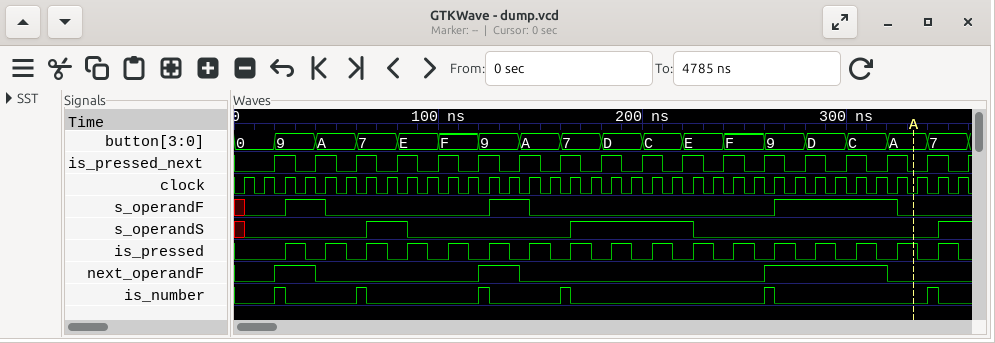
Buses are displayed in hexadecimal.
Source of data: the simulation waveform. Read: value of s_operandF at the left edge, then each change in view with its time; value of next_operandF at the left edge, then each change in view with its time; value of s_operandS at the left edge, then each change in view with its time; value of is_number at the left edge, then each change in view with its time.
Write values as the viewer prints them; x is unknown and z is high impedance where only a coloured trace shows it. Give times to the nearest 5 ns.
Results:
x, 0 at 5 ns, 1 at 25 ns, 0 at 45 ns, 1 at 125 ns, 0 at 145 ns, 1 at 265 ns, 0 at 325 ns
0, 1 at 20 ns, 0 at 40 ns, 1 at 120 ns, 0 at 140 ns, 1 at 260 ns, 0 at 320 ns
x, 0 at 5 ns, 1 at 65 ns, 0 at 85 ns, 1 at 165 ns, 0 at 225 ns, 1 at 345 ns
0, 1 at 20 ns, 0 at 25 ns, 1 at 60 ns, 0 at 65 ns, 1 at 120 ns, 0 at 125 ns, 1 at 160 ns, 0 at 165 ns, 1 at 260 ns, 0 at 265 ns, 1 at 340 ns, 0 at 345 ns
